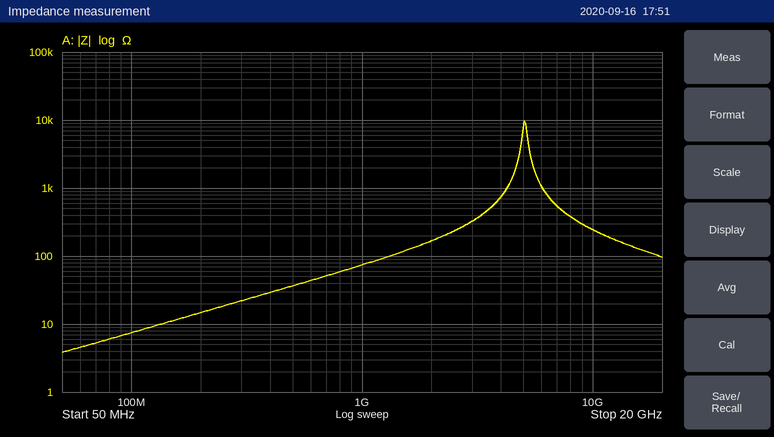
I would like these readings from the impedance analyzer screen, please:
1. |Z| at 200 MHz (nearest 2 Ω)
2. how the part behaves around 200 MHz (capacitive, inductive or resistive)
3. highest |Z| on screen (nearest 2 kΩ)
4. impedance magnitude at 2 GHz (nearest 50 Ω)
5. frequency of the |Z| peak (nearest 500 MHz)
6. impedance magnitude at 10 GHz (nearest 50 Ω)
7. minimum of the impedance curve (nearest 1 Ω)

14 Ω
inductive
10 kΩ
150 Ω
5.0 GHz
250 Ω
4 Ω
